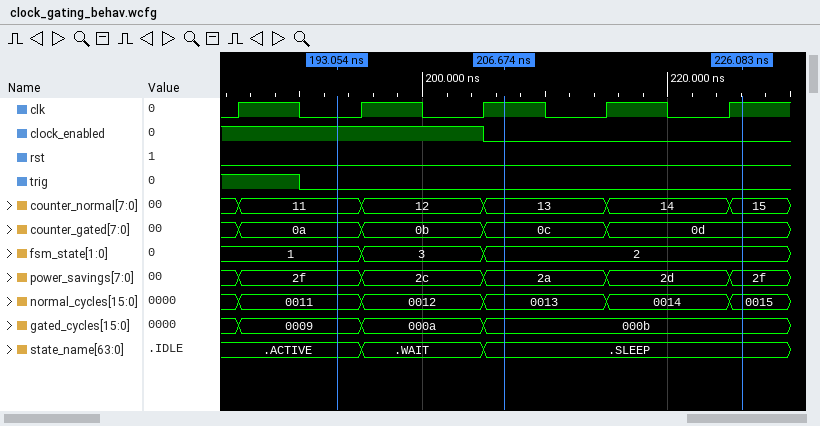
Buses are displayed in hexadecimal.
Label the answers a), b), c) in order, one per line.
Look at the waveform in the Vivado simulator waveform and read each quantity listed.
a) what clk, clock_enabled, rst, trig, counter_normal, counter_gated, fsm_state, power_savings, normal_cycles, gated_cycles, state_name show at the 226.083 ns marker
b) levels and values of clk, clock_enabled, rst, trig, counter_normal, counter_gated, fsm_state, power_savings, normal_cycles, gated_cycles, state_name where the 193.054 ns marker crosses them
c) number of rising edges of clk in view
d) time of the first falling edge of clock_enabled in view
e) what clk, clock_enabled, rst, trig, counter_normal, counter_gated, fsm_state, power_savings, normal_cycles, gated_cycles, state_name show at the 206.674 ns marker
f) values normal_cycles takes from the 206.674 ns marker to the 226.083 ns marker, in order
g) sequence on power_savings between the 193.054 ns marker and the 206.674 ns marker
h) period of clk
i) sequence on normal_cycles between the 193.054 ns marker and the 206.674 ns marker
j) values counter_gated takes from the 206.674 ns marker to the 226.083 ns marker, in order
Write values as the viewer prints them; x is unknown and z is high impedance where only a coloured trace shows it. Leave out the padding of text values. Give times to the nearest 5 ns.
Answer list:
a) clk=1, clock_enabled=0, rst=0, trig=0, counter_normal=15, counter_gated=0d, fsm_state=2, power_savings=2f, normal_cycles=0015, gated_cycles=000b, state_name=SLEEP
b) clk=0, clock_enabled=1, rst=0, trig=0, counter_normal=11, counter_gated=0a, fsm_state=1, power_savings=2f, normal_cycles=0011, gated_cycles=0009, state_name=ACTIVE
c) 5
d) 205 ns
e) clk=1, clock_enabled=0, rst=0, trig=0, counter_normal=13, counter_gated=0c, fsm_state=2, power_savings=2a, normal_cycles=0013, gated_cycles=000b, state_name=SLEEP
f) 0013, 0014, 0015
g) 2f, 2c, 2a
h) 10 ns
i) 0011, 0012, 0013
j) 0c, 0d
